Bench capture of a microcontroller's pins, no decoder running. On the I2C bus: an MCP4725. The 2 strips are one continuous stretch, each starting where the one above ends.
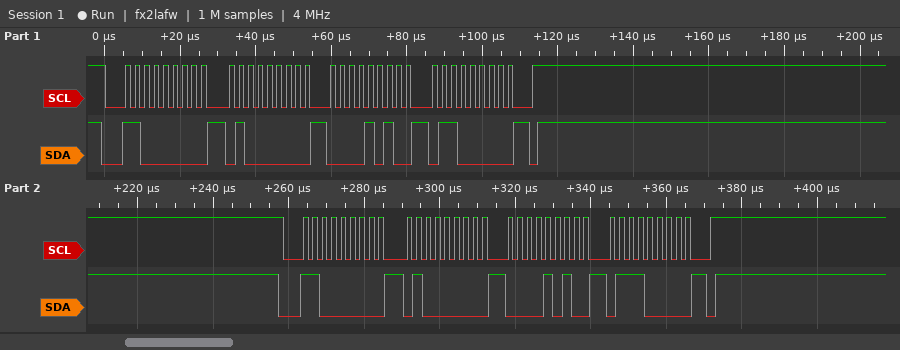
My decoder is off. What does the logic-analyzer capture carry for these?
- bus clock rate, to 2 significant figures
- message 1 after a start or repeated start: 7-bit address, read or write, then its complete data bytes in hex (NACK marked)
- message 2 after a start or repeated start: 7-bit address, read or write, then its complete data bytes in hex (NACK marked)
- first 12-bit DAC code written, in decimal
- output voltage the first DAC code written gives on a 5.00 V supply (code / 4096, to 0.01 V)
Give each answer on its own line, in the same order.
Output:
400 kHz
0x60 write: 40 0A 60
0x60 write: 40 0A 70
166
0.20 V
